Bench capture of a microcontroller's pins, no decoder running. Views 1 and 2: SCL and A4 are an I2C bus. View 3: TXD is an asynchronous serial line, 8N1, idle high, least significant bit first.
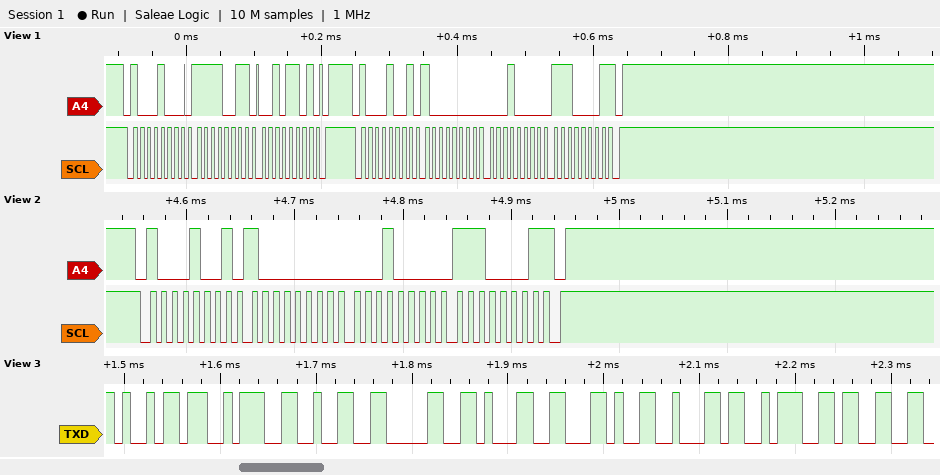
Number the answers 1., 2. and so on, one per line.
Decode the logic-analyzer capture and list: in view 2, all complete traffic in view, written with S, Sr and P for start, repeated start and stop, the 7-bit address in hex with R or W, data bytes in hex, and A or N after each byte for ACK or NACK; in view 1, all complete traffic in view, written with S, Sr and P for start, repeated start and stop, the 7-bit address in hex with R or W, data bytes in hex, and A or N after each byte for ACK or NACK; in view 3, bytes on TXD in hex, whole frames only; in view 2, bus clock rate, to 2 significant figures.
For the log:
1. S 44R A 80 A 10 A E1 N P
2. S 44W A F3 A 2D A P S 44R A 80 A 10 A E1 N P
3. 0x69 0x3A 0x32 0x30 0x31 0x2C 0x62 0x3A 0x33
4. 100 kHz
